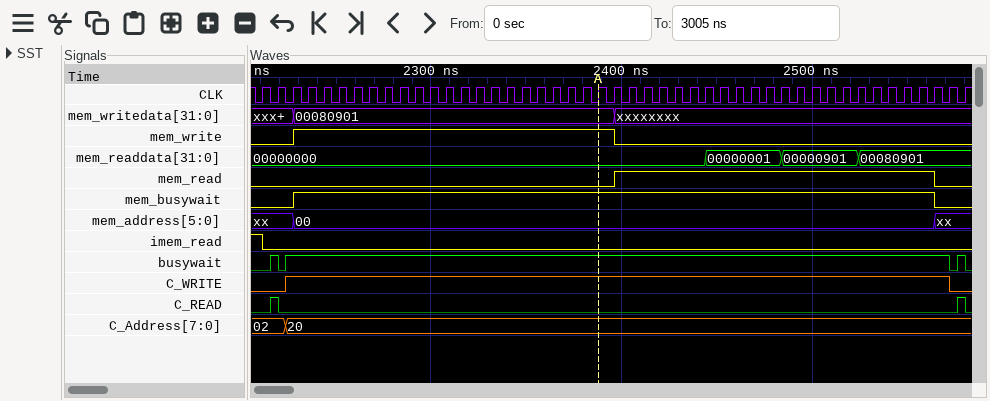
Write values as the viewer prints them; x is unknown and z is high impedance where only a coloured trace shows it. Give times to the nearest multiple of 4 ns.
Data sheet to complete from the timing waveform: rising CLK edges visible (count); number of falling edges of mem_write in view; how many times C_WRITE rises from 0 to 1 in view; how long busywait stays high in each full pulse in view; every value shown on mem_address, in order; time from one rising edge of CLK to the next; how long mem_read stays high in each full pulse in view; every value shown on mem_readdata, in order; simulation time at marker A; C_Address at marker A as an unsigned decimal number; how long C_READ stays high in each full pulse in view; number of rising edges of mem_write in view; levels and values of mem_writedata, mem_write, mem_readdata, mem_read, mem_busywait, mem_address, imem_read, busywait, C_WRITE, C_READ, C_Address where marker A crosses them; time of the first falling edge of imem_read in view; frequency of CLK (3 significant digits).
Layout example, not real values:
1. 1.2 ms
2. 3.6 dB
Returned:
1. 47
2. 1
3. 1
4. 4 ns, 348 ns, 4 ns
5. xx, 00, xx
6. 8 ns
7. 168 ns
8. 00000000, 00000001, 00000901, 00080901
9. 2388 ns
10. 32
11. 4 ns, 4 ns
12. 1
13. mem_writedata=00080901, mem_write=1, mem_readdata=00000000, mem_read=0, mem_busywait=1, mem_address=00, imem_read=0, busywait=1, C_WRITE=1, C_READ=0, C_Address=20
14. 2212 ns
15. 125 MHz
